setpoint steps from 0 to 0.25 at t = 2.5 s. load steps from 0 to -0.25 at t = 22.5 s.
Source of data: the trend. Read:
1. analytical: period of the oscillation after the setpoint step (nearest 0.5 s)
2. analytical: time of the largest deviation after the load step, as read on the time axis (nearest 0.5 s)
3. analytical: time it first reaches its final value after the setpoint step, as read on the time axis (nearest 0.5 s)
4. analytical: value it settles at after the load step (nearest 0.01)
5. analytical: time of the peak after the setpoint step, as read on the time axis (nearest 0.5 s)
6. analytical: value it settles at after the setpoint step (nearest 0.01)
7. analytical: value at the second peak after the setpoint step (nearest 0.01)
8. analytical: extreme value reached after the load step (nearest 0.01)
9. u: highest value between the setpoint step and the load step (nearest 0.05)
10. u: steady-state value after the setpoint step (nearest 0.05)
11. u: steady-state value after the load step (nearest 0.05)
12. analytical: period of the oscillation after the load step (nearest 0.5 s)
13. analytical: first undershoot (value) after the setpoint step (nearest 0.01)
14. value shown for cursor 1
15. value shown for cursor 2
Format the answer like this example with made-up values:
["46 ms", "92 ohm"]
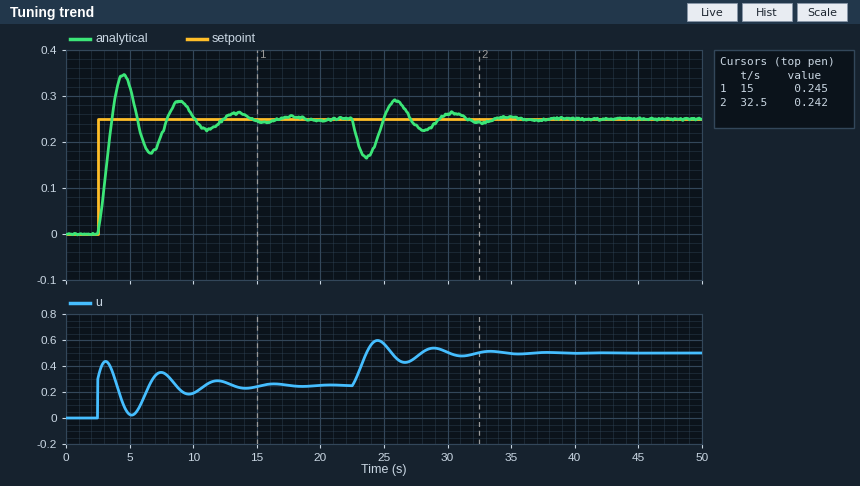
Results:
["4.5 s", "23.5 s", "3.5 s", "0.25", "4.5 s", "0.25", "0.29", "0.17", "0.45", "0.25", "0.50", "4.5 s", "0.18", "0.245", "0.242"]
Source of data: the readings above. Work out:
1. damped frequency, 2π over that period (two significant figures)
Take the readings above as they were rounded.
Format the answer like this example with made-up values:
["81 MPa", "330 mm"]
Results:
["1.4 rad/s"]
